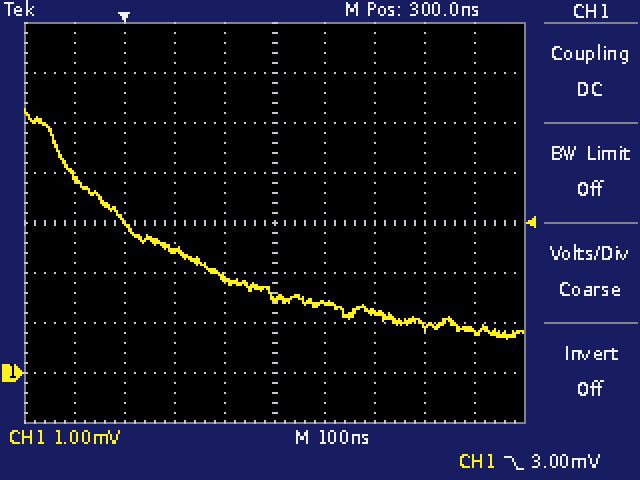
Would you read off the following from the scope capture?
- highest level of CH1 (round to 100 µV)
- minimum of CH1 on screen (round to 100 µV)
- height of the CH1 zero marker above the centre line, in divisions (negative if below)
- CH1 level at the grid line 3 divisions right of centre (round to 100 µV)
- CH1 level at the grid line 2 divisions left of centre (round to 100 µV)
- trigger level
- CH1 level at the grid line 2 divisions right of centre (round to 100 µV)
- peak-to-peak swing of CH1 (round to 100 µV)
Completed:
5.3 mV
700 µV
-3.0 div
900 µV
2.4 mV
3.00 mV
1.2 mV
4.6 mV
